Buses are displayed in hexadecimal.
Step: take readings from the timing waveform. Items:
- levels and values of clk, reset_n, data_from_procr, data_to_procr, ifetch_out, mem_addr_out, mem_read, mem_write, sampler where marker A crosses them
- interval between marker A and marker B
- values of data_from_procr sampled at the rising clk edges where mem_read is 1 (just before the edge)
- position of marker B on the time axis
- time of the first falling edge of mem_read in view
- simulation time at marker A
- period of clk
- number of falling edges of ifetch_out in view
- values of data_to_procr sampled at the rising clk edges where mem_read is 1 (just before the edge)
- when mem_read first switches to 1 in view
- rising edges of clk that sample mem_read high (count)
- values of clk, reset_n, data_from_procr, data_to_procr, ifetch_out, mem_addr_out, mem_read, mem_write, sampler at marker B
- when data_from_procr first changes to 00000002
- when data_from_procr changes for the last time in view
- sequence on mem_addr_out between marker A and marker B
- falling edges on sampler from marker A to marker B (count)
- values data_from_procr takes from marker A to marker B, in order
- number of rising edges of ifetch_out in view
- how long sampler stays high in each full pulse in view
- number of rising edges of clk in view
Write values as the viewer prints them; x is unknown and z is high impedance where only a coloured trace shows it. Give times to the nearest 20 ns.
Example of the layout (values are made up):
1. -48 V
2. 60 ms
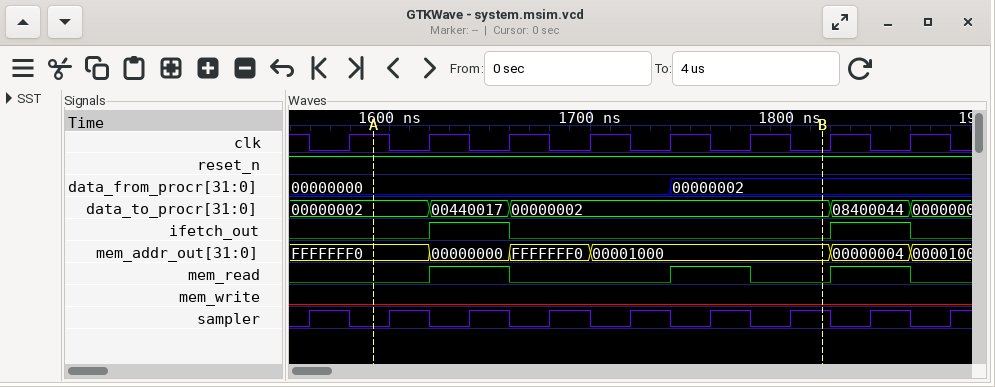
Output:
1. clk=1, reset_n=1, data_from_procr=00000000, data_to_procr=00000002, ifetch_out=0, mem_addr_out=FFFFFFF0, mem_read=0, mem_write=0, sampler=0
2. 220 ns
3. 00000000, 00000002, 00000002
4. 1820 ns
5. 1660 ns
6. 1600 ns
7. 40 ns
8. 2
9. 00440017, 00000002, 08400044
10. 1620 ns
11. 3
12. clk=0, reset_n=1, data_from_procr=00000002, data_to_procr=00000002, ifetch_out=0, mem_addr_out=00001000, mem_read=0, mem_write=0, sampler=1
13. 1740 ns
14. 1740 ns
15. FFFFFFF0, 00000000, FFFFFFF0, 00001000
16. 5
17. 00000000, 00000002
18. 2
19. 20 ns, 20 ns, 20 ns, 20 ns, 20 ns, 20 ns, 20 ns, 20 ns
20. 8
